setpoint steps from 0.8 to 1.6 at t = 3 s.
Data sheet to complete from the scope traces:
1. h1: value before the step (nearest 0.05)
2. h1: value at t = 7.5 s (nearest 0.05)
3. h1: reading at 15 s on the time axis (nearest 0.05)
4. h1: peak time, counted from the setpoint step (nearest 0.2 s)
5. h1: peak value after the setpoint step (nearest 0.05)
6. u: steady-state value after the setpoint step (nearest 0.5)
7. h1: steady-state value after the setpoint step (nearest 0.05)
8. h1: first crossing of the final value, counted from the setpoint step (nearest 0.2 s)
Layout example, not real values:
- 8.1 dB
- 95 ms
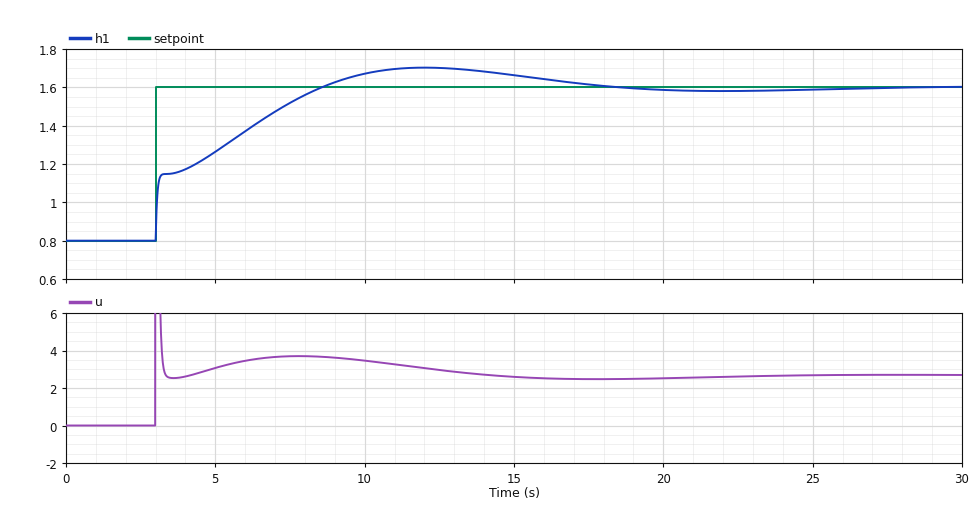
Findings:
- 0.80
- 1.50
- 1.65
- 9.0 s
- 1.70
- 2.5
- 1.60
- 5.6 s
